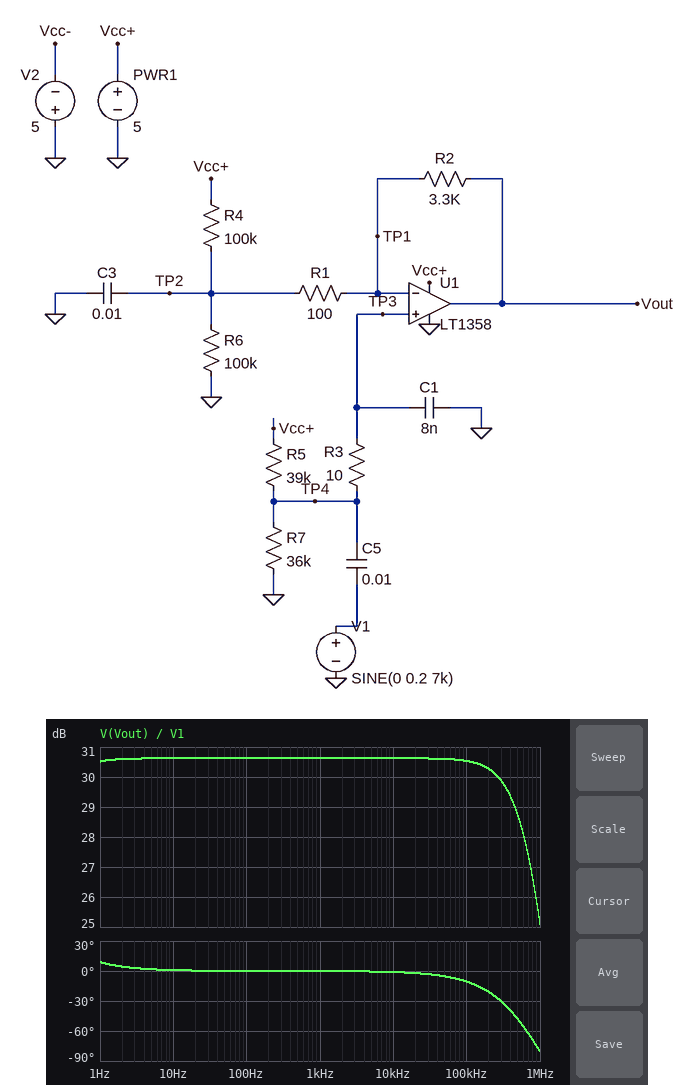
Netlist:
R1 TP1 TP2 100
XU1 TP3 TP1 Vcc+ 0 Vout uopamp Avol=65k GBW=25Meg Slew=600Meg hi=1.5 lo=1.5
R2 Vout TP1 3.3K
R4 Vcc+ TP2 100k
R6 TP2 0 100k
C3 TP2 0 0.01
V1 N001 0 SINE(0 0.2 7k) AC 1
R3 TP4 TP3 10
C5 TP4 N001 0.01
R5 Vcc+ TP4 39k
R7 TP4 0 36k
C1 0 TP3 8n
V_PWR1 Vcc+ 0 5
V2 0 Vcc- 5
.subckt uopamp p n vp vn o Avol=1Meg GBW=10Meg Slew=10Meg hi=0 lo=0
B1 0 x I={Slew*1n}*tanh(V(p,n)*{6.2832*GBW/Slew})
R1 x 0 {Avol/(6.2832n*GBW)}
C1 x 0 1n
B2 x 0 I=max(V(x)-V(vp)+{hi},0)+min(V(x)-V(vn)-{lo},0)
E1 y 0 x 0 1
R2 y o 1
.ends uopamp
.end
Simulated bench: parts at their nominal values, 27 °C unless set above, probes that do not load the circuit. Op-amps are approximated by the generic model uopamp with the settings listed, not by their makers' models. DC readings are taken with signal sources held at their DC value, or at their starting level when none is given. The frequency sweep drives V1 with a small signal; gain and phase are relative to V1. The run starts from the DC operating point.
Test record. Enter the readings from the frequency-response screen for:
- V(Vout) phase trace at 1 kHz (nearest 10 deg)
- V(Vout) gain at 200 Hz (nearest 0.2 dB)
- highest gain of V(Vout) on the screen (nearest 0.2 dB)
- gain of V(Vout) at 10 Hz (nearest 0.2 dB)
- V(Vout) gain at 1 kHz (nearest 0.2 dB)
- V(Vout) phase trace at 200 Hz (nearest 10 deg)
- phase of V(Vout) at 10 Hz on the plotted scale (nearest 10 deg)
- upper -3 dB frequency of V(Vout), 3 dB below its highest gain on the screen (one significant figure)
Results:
0 deg
30.6 dB
30.6 dB
30.6 dB
30.6 dB
0 deg
0 deg
700 kHz
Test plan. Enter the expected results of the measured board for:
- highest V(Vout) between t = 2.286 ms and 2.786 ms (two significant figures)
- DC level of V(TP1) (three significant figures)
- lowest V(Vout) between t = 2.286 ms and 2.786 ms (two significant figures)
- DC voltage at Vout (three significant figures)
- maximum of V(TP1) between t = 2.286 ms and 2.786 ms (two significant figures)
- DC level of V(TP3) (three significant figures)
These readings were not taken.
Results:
3.5 V
2.40 V
1.5 V
2.39 V
2.4 V
2.40 V
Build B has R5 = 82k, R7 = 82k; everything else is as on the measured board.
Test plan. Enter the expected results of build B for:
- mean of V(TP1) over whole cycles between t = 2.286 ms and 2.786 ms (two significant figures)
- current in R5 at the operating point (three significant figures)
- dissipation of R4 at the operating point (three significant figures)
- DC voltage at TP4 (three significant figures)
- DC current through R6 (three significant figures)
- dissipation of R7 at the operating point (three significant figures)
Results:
2.5 V
30.5 µA
62.5 µW
2.50 V
25.0 µA
76.2 µW
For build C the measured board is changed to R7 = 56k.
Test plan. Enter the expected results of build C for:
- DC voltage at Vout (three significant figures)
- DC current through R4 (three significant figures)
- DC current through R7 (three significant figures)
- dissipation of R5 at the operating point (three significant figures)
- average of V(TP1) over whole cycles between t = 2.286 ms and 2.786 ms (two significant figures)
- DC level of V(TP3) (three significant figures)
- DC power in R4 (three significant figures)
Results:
2.98 V
20.5 µA
52.6 µA
108 µW
2.9 V
2.95 V
42.2 µW
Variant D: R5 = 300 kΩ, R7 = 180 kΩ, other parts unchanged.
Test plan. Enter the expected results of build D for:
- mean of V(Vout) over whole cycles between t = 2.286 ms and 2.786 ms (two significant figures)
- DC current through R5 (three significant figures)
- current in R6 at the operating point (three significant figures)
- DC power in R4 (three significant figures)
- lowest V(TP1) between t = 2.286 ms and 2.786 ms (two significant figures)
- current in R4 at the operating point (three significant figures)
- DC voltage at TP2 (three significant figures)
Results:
2.4 V
10.4 µA
18.8 µA
97.6 µW
1.9 V
31.2 µA
1.88 V
